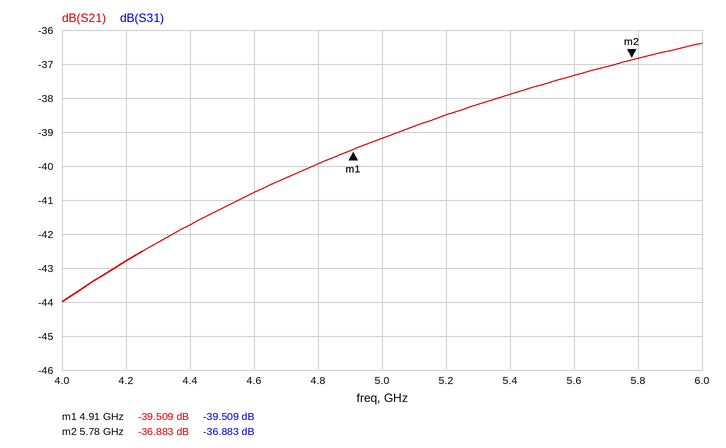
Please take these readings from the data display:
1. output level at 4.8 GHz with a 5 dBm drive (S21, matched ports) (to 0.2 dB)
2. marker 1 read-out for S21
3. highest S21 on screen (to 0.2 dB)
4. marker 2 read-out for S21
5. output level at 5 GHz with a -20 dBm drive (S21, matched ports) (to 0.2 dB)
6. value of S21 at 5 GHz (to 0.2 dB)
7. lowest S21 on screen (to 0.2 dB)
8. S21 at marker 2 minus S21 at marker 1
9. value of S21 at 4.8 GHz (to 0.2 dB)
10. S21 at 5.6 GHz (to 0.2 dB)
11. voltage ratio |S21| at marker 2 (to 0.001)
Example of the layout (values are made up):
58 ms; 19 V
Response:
-35.0 dBm; -39.509 dB; -36.4 dB; -36.883 dB; -59.2 dBm; -39.2 dB; -44.0 dB; 2.626 dB; -40.0 dB; -37.4 dB; 0.014
